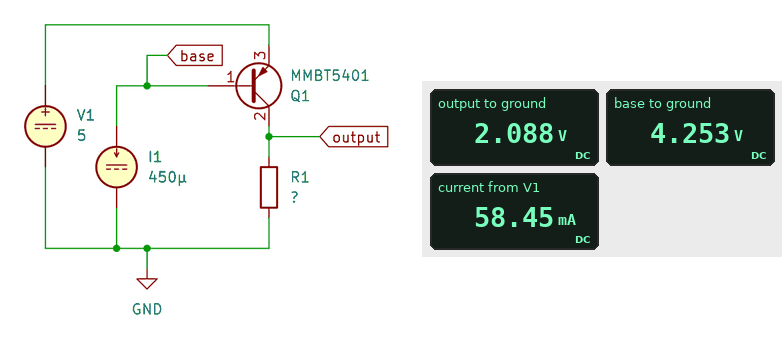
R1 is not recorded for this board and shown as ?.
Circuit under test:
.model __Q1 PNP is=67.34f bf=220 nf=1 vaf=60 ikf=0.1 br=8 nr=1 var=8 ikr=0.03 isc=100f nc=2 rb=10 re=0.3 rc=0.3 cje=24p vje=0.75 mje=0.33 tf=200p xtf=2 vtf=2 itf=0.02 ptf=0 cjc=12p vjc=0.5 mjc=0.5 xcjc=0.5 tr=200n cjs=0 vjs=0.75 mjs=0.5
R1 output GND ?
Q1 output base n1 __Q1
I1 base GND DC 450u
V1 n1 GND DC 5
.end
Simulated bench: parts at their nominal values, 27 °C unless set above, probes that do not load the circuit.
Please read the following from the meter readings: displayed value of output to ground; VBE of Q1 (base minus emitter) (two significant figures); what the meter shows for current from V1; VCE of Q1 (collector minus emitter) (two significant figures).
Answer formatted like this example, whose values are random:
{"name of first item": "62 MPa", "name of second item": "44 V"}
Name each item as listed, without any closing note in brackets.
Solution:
{"displayed value of output to ground": "2.088 V", "VBE of Q1 (base minus emitter)": "-750 mV", "what the meter shows for current from V1": "58.45 mA", "VCE of Q1 (collector minus emitter)": "-2.9 V"}
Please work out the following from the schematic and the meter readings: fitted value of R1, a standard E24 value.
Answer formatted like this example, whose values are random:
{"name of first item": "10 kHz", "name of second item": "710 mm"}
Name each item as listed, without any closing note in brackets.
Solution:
{"fitted value of R1, a standard E24 value": "36 Ω"}
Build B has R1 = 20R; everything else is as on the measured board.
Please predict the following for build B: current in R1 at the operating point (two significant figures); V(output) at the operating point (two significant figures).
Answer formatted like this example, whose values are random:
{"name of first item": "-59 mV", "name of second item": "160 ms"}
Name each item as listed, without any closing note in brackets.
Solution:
{"current in R1 at the operating point": "59 mA", "V(output) at the operating point": "1.2 V"}
